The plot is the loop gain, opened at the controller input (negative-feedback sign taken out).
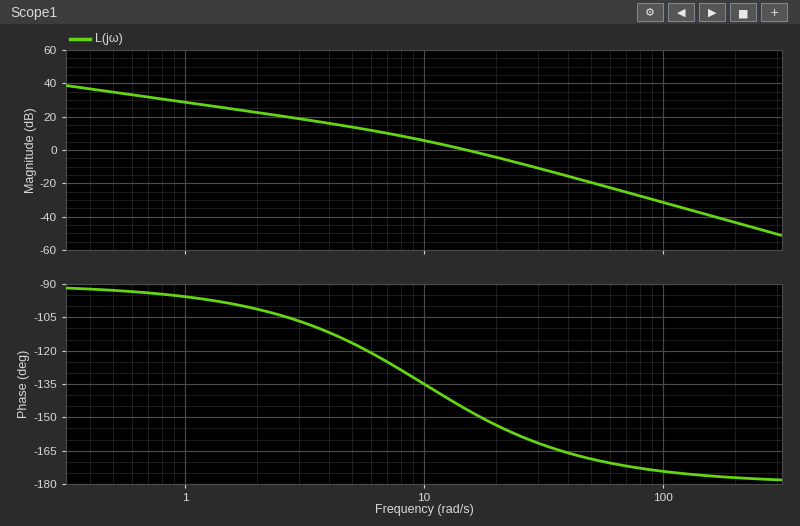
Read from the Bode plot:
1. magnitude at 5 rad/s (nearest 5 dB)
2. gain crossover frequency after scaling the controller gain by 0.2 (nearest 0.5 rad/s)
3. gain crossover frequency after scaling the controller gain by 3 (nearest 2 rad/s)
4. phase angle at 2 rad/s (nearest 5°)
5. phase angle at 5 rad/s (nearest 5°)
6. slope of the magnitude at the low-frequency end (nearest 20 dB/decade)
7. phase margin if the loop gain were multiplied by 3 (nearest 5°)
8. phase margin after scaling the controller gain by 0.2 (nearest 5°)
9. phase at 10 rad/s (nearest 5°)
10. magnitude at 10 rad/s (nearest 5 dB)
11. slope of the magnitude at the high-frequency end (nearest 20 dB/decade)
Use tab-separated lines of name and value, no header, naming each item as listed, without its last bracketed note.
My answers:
magnitude at 5 rad/s	15 dB
gain crossover frequency after scaling the controller gain by 0.2	5.0 rad/s
gain crossover frequency after scaling the controller gain by 3	28 rad/s
phase angle at 2 rad/s	-100°
phase angle at 5 rad/s	-115°
slope of the magnitude at the low-frequency end	-20 dB/decade
phase margin if the loop gain were multiplied by 3	20°
phase margin after scaling the controller gain by 0.2	65°
phase at 10 rad/s	-135°
magnitude at 10 rad/s	5 dB
slope of the magnitude at the high-frequency end	-40 dB/decade
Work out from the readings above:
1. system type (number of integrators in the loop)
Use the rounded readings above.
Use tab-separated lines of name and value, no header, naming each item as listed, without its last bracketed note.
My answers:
system type	1
